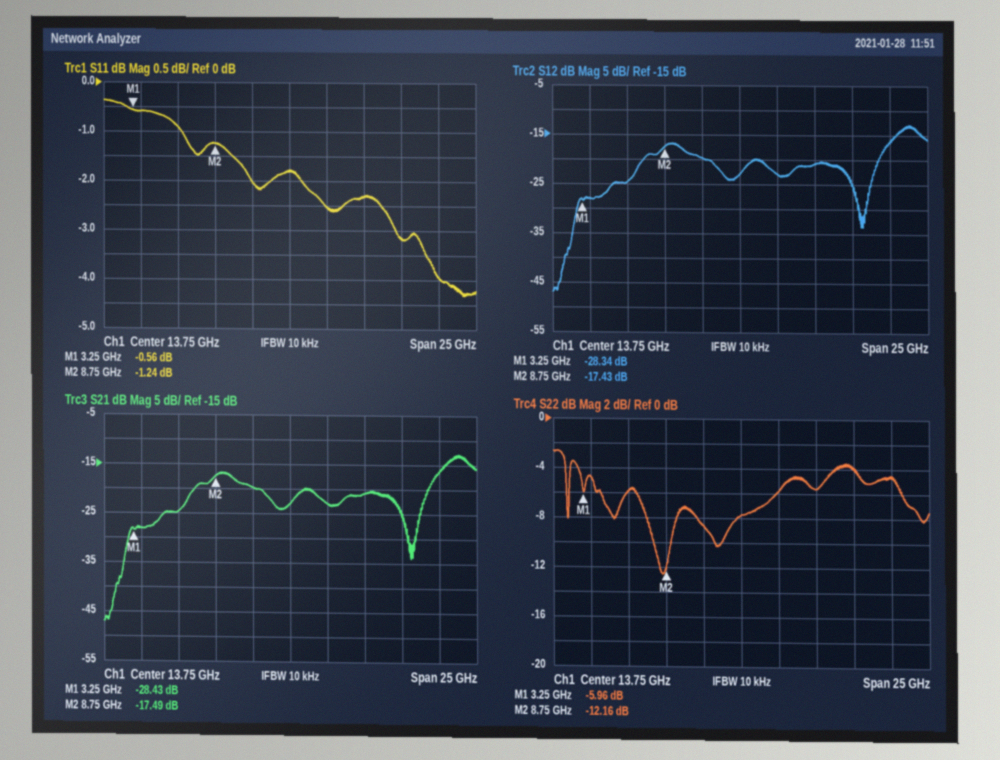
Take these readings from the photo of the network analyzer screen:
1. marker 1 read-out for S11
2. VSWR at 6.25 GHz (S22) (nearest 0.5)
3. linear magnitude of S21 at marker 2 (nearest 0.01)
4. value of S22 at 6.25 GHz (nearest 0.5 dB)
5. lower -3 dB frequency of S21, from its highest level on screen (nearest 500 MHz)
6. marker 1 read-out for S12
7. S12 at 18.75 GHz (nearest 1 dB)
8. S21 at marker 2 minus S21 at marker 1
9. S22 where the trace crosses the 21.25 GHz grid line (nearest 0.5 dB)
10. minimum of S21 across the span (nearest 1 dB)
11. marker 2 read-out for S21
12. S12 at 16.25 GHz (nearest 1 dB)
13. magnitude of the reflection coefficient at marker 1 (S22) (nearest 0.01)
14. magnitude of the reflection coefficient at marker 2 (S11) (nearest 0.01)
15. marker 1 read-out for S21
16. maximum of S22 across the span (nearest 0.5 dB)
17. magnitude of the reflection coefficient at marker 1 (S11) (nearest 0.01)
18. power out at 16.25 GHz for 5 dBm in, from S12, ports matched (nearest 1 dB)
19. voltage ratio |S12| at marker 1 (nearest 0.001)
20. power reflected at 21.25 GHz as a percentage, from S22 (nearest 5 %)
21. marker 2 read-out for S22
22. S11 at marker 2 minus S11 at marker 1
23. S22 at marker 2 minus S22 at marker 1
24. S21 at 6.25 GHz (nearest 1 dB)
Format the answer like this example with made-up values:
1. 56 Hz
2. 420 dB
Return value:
1. -0.56 dB
2. 3.0
3. 0.13
4. -6.0 dB
5. 24.0 GHz
6. -28.34 dB
7. -21 dB
8. 10.94 dB
9. -4.0 dB
10. -47 dB
11. -17.49 dB
12. -23 dB
13. 0.50
14. 0.87
15. -28.43 dB
16. -2.5 dB
17. 0.94
18. -18 dBm
19. 0.038
20. 40 %
21. -12.16 dB
22. -0.68 dB
23. -6.20 dB
24. -25 dB
